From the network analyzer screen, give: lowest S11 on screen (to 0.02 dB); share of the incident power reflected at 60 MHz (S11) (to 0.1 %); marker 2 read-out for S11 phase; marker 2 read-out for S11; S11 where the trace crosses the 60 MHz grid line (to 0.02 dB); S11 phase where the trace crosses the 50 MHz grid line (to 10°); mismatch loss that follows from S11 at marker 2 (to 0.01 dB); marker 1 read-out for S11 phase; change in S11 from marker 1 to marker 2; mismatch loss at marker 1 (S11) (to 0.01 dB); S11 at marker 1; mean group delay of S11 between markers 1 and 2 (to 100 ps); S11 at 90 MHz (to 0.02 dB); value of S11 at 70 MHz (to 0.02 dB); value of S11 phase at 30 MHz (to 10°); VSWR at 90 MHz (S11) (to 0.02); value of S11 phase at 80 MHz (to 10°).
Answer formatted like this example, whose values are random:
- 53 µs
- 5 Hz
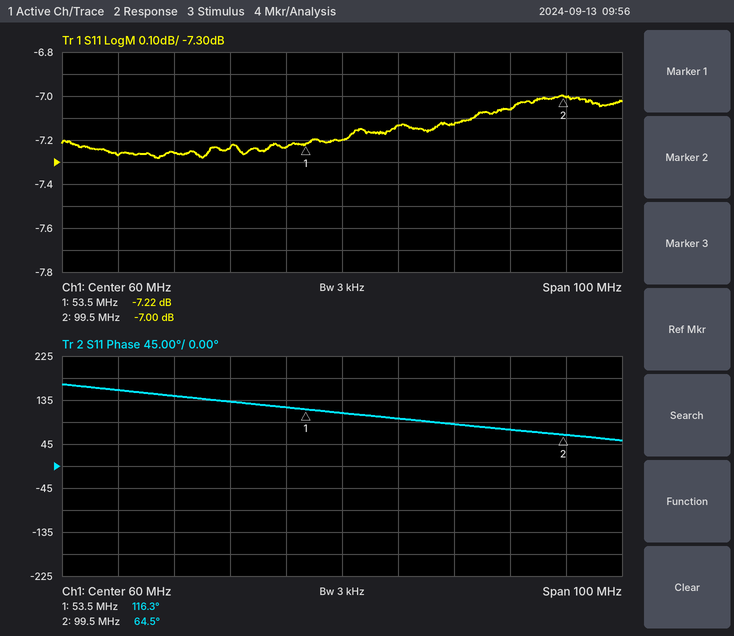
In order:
- -7.28 dB
- 19.1 %
- 64.5°
- -7.00 dB
- -7.20 dB
- 120°
- 0.97 dB
- 116.3°
- 0.22 dB
- 0.91 dB
- -7.22 dB
- 3.1 ns
- -7.06 dB
- -7.14 dB
- 140°
- 2.60
- 90°
